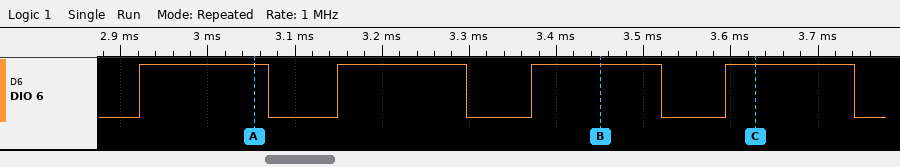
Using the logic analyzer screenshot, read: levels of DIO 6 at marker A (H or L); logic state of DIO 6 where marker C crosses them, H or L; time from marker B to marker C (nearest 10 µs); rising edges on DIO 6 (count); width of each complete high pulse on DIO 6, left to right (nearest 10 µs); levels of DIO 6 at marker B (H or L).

DIO 6=H
DIO 6=H
180 µs
4
150 µs, 150 µs, 150 µs, 150 µs
DIO 6=H
